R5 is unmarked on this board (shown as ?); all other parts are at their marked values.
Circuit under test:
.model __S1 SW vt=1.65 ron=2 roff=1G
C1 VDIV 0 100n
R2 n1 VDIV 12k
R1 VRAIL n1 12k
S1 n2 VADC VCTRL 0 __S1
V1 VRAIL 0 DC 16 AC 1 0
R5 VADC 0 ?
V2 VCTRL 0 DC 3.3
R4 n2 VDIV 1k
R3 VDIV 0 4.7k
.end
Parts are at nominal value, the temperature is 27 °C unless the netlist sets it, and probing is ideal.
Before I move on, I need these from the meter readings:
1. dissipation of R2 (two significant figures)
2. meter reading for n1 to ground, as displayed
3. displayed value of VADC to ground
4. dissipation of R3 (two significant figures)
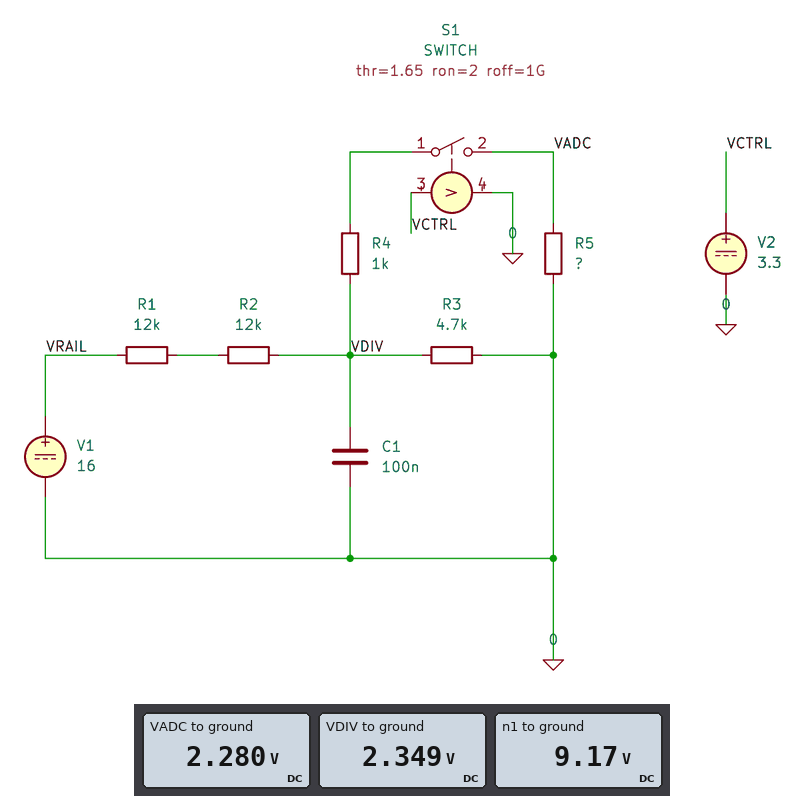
3.9 mW
9.17 V
2.280 V
1.2 mW
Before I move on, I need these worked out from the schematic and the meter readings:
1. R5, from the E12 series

33 kΩ
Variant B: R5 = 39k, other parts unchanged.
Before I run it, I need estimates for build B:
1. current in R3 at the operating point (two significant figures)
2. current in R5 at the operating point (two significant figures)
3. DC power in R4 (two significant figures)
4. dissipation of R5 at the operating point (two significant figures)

510 µA
60 µA
3.6 µW
140 µW
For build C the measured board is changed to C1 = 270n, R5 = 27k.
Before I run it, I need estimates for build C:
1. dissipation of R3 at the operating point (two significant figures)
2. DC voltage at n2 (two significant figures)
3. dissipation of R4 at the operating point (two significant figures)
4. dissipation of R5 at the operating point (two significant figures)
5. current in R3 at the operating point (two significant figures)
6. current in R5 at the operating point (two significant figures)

1.1 mW
2.2 V
6.7 µW
180 µW
490 µA
82 µA
